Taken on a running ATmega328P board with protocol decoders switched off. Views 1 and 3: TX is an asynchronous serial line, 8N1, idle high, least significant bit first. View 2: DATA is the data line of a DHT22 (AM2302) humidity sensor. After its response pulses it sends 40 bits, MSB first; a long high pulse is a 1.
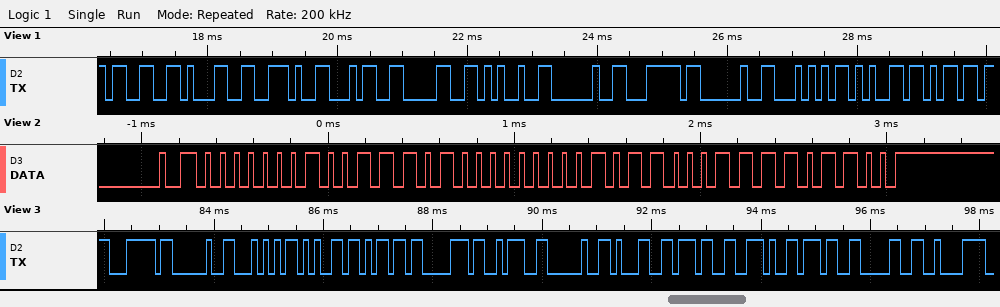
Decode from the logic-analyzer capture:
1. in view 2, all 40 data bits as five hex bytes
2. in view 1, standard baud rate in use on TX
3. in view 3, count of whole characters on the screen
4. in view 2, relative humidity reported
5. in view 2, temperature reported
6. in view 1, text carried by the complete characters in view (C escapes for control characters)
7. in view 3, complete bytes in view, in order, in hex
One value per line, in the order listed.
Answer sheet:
01 3A 00 B1 EC
9600 baud
14
31.4 %
17.7 °C
"31.40% | Tem"
7C 20 54 65 6D 70 3A 20 31 37 2E 37 30 C2
